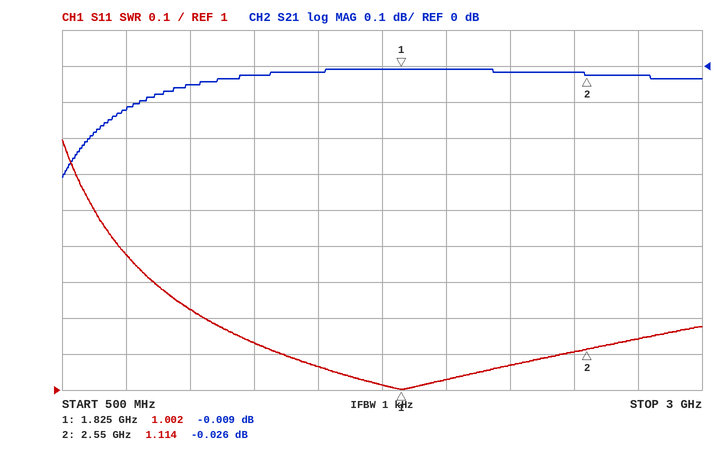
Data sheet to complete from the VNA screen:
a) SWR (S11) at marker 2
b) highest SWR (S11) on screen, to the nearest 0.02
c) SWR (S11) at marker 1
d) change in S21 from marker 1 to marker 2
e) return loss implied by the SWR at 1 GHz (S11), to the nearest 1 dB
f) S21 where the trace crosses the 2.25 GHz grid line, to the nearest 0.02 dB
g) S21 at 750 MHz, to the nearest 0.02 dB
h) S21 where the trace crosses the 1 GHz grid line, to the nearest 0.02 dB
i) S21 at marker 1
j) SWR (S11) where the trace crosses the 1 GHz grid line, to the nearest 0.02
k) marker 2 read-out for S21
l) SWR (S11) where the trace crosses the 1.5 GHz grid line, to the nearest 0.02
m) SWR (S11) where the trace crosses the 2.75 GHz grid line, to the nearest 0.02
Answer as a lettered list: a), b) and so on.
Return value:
a) 1.114
b) 1.70
c) 1.002
d) -0.017 dB
e) 20 dB
f) -0.02 dB
g) -0.12 dB
h) -0.06 dB
i) -0.009 dB
j) 1.22
k) -0.026 dB
l) 1.06
m) 1.14
